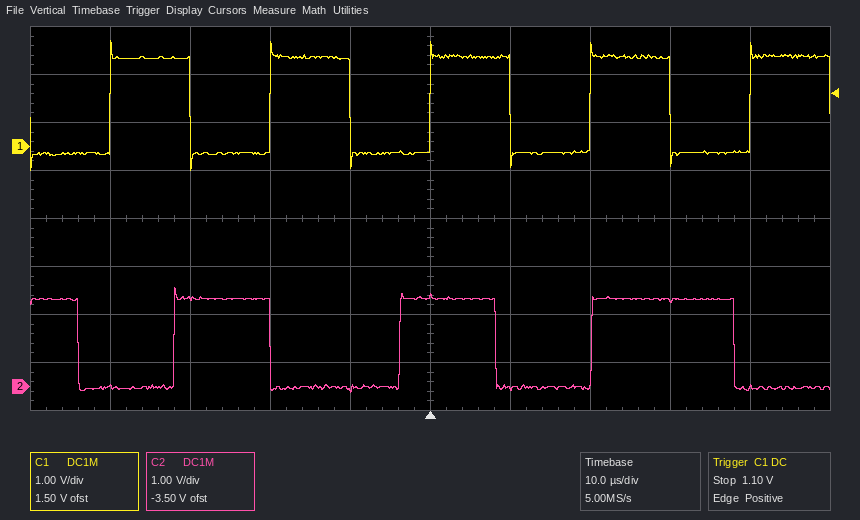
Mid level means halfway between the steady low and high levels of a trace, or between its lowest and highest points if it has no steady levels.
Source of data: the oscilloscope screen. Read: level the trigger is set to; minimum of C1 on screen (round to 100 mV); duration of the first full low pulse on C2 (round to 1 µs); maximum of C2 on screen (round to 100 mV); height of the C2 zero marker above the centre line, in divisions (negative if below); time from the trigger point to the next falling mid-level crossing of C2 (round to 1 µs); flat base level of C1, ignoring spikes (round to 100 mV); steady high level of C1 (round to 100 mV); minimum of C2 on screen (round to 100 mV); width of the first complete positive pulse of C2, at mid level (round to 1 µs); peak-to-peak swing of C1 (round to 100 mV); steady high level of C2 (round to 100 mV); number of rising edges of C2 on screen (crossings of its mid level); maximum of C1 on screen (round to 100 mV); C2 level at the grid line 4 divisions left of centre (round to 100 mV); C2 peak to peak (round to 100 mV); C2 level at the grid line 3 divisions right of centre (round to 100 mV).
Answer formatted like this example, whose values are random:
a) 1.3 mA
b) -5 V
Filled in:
a) 1.10 V
b) -500 mV
c) 12 µs
d) 2.1 V
e) -3.5 div
f) 8 µs
g) -100 mV
h) 1.9 V
i) -100 mV
j) 12 µs
k) 2.7 V
l) 1.8 V
m) 3
n) 2.2 V
o) 0.0 V
p) 2.2 V
q) 1.8 V
